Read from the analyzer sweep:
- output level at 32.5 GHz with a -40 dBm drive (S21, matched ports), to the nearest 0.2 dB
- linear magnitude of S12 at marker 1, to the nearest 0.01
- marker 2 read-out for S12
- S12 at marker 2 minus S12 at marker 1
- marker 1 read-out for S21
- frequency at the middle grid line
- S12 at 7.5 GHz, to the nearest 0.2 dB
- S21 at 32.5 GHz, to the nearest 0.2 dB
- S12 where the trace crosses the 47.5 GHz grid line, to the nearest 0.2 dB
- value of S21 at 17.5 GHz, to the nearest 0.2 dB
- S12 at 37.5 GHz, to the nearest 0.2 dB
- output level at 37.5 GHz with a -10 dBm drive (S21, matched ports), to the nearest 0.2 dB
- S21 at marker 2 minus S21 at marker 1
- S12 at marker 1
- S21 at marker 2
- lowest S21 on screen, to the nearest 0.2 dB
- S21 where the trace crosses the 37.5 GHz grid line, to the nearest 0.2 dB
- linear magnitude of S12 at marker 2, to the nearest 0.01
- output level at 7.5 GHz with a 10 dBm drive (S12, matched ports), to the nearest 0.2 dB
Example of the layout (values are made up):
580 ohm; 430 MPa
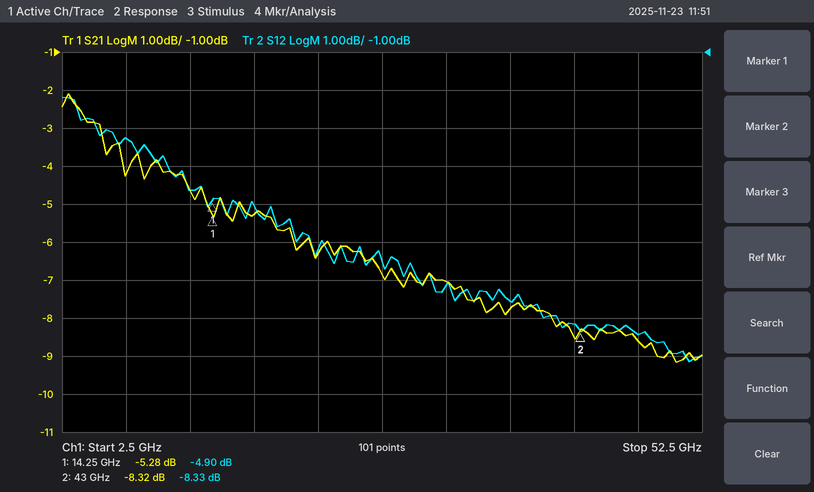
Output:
-47.0 dBm; 0.57; -8.33 dB; -3.43 dB; -5.28 dB; 27.5 GHz; -3.2 dB; -7.0 dB; -8.4 dB; -5.2 dB; -7.6 dB; -17.8 dBm; -3.04 dB; -4.90 dB; -8.32 dB; -9.2 dB; -7.8 dB; 0.38; 6.8 dBm
